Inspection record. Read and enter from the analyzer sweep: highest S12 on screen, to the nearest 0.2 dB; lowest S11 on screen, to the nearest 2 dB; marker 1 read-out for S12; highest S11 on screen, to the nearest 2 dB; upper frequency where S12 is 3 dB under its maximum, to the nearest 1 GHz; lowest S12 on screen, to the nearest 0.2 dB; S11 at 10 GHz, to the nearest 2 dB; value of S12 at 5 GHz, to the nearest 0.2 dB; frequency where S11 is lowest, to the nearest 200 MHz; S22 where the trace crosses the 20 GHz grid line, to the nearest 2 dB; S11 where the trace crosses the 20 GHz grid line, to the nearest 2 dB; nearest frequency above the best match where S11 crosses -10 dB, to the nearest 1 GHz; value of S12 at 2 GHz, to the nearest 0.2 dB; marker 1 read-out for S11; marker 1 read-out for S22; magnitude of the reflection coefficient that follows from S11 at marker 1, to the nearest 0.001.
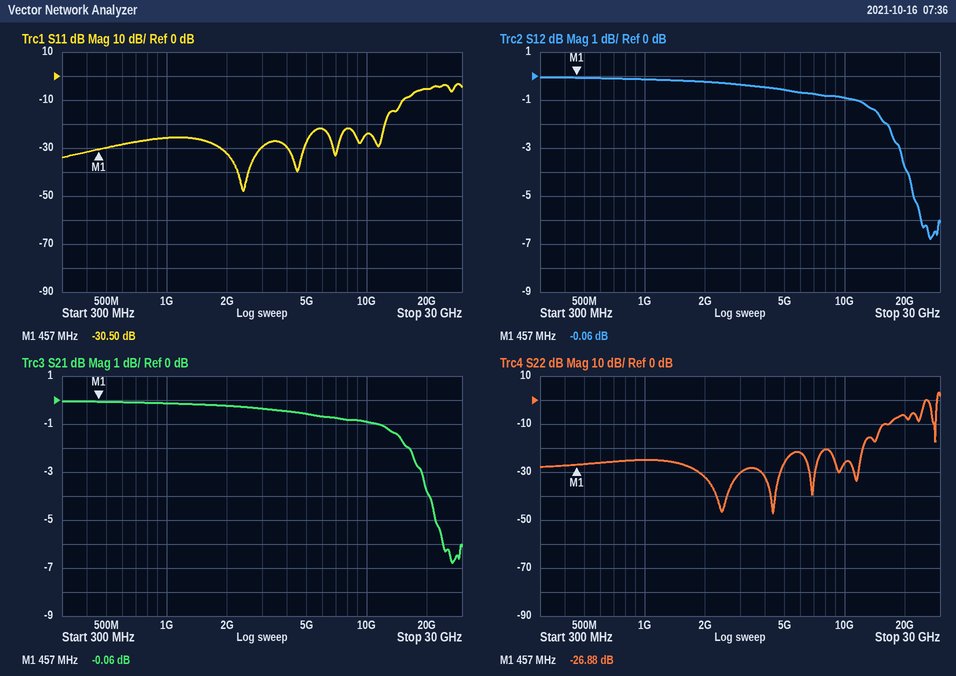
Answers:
0.0 dB
-48 dB
-0.06 dB
-4 dB
19 GHz
-6.8 dB
-24 dB
-0.6 dB
2.4 GHz
-6 dB
-6 dB
15 GHz
-0.2 dB
-30.50 dB
-26.88 dB
0.030
